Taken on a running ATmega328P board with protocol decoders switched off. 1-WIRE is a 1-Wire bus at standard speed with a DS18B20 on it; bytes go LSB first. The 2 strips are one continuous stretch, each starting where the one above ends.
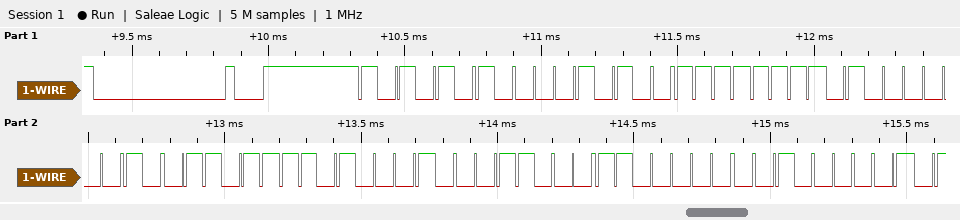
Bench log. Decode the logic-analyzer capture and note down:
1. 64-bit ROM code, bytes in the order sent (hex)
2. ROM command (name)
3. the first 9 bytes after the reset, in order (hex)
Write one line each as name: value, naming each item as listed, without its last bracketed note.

64-bit ROM code, bytes in the order sent: 28 FF 02 D9 8B 18 03 82
ROM command: Match ROM
the first 9 bytes after the reset, in order: 55 28 FF 02 D9 8B 18 03 82
